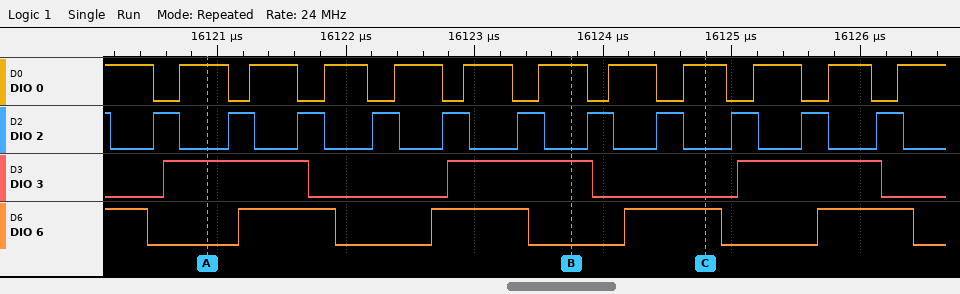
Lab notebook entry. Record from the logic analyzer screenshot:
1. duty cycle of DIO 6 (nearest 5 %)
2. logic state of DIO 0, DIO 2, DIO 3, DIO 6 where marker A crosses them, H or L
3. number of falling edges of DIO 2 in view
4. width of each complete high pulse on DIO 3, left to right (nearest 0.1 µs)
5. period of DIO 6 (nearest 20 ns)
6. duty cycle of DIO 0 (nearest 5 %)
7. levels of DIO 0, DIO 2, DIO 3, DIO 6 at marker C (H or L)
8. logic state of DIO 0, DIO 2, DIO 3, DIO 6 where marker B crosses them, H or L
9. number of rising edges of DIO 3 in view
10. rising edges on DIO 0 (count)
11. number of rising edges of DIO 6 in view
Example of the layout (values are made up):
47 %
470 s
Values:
50 %
DIO 0=H, DIO 2=L, DIO 3=H, DIO 6=L
12
1.1 µs, 1.1 µs, 1.1 µs
1500 ns
65 %
DIO 0=H, DIO 2=L, DIO 3=L, DIO 6=H
DIO 0=H, DIO 2=L, DIO 3=H, DIO 6=L
3
11
4
